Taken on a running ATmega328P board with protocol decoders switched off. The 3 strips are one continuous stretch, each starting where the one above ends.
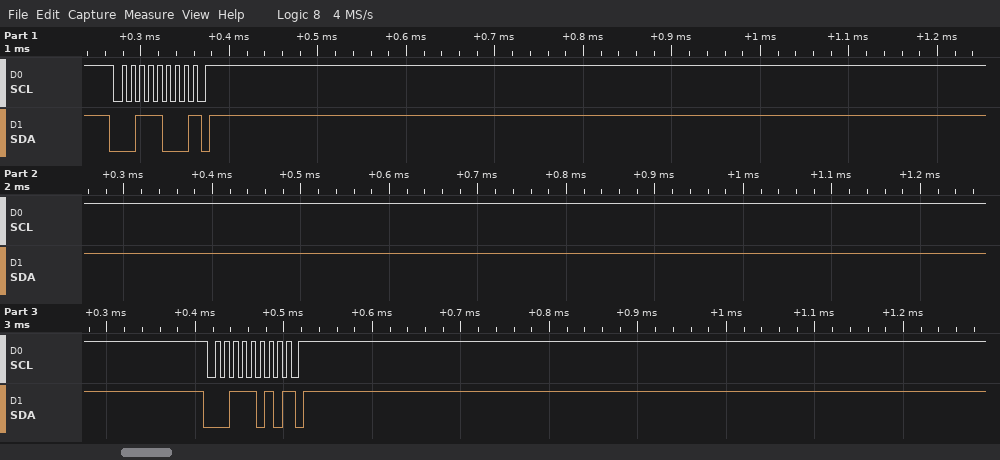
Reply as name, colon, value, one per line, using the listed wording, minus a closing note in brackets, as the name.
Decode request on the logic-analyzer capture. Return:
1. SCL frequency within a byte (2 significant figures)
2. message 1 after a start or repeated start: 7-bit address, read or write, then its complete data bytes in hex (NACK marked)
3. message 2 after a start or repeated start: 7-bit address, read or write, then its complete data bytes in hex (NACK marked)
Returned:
SCL frequency within a byte: 100 kHz
message 1 after a start or repeated start: 7-bit address, read or write, then its complete data bytes in hex: 0x1C write NACK
message 2 after a start or repeated start: 7-bit address, read or write, then its complete data bytes in hex: 0x1D write NACK
